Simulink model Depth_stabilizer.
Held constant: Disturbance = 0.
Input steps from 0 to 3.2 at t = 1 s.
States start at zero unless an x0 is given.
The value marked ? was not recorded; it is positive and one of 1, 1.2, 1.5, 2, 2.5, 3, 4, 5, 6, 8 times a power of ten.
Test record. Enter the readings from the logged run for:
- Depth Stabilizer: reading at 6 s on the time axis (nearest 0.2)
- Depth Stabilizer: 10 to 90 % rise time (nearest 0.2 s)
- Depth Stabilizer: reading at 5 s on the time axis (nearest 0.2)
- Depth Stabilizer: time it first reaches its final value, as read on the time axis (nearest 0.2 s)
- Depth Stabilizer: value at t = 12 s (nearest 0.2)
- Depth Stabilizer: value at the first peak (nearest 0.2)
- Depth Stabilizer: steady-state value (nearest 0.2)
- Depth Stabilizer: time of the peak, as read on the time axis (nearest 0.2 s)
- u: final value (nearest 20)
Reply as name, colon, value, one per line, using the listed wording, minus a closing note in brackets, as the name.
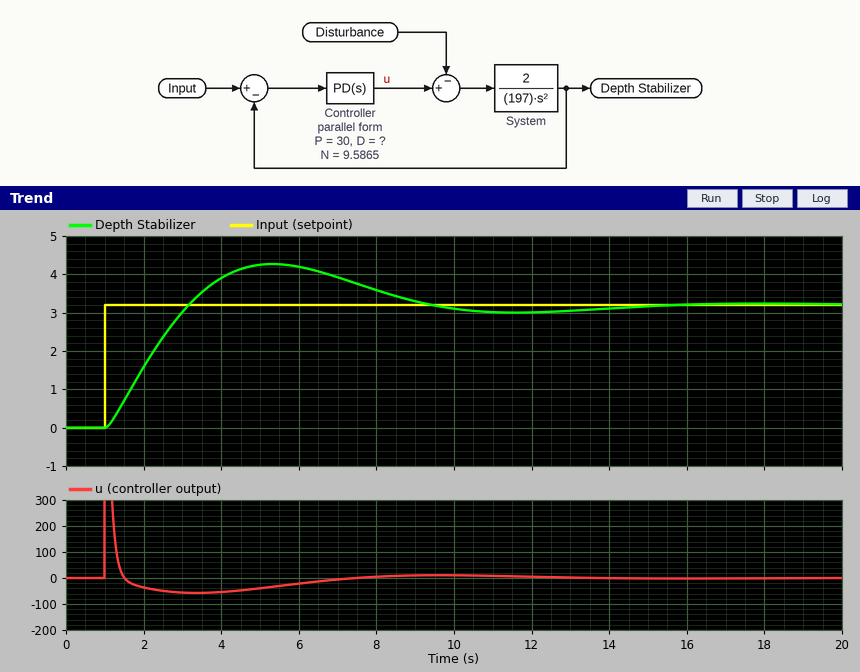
Depth Stabilizer: reading at 6 s on the time axis: 4.2
Depth Stabilizer: 10 to 90 % rise time: 1.6 s
Depth Stabilizer: reading at 5 s on the time axis: 4.2
Depth Stabilizer: time it first reaches its final value, as read on the time axis: 3.2 s
Depth Stabilizer: value at t = 12 s: 3.0
Depth Stabilizer: value at the first peak: 4.2
Depth Stabilizer: steady-state value: 3.2
Depth Stabilizer: time of the peak, as read on the time axis: 5.4 s
u: final value: 0
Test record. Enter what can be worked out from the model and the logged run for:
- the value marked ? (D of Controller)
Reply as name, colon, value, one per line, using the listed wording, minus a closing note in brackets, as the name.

the value marked ?: 50
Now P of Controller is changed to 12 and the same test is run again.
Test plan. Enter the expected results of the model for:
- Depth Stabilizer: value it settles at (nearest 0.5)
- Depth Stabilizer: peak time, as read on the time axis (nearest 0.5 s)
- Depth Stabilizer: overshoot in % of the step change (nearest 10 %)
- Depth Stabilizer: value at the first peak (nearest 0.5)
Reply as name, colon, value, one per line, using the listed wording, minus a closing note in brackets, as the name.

Depth Stabilizer: value it settles at: 3.0
Depth Stabilizer: peak time, as read on the time axis: 7.0 s
Depth Stabilizer: overshoot in % of the step change: 20 %
Depth Stabilizer: value at the first peak: 4.0
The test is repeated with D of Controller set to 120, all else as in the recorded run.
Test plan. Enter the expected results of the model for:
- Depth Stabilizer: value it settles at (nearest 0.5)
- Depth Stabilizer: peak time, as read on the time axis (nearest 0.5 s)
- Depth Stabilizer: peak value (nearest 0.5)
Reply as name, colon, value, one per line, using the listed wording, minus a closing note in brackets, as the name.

Depth Stabilizer: value it settles at: 3.0
Depth Stabilizer: peak time, as read on the time axis: 4.0 s
Depth Stabilizer: peak value: 3.5
